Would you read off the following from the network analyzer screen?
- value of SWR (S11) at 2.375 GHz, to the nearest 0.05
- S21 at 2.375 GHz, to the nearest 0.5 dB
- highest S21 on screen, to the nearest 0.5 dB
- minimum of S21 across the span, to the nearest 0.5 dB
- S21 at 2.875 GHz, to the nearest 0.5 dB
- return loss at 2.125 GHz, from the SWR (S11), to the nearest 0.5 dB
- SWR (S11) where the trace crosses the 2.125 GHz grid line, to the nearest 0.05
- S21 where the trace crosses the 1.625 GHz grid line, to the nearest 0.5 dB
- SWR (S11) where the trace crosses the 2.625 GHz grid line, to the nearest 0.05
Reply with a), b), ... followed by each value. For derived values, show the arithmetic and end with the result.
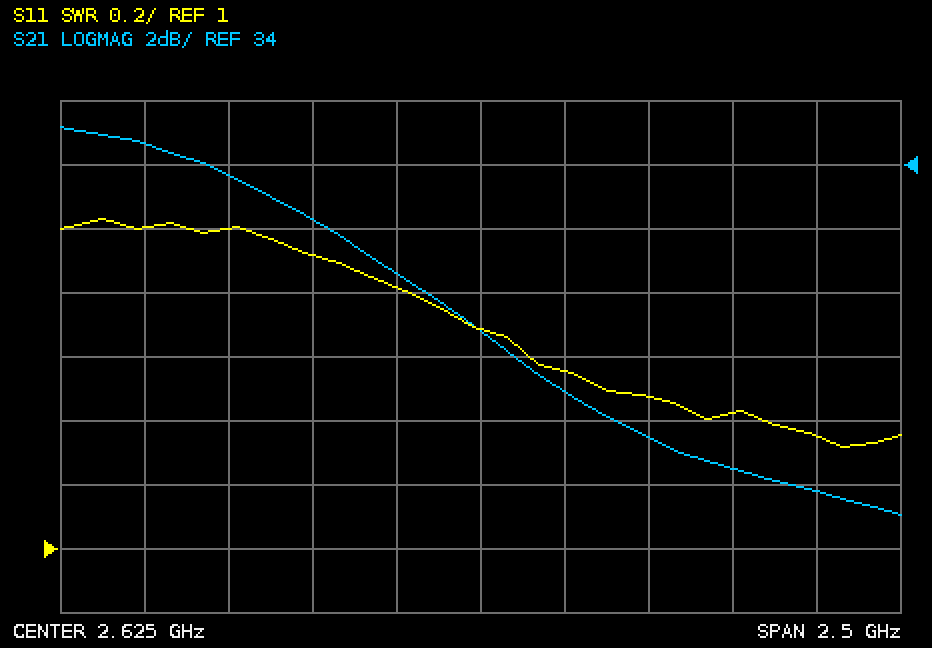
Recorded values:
a) 1.80
b) 30.5 dB
c) 35.0 dB
d) 23.0 dB
e) 27.0 dB
f) −20 log10((1.9 − 1)/(1.9 + 1)) ≈ 10.2 dB, so 10.0 dB to the nearest 0.5 dB
g) 1.90
h) 34.5 dB
i) 1.70
